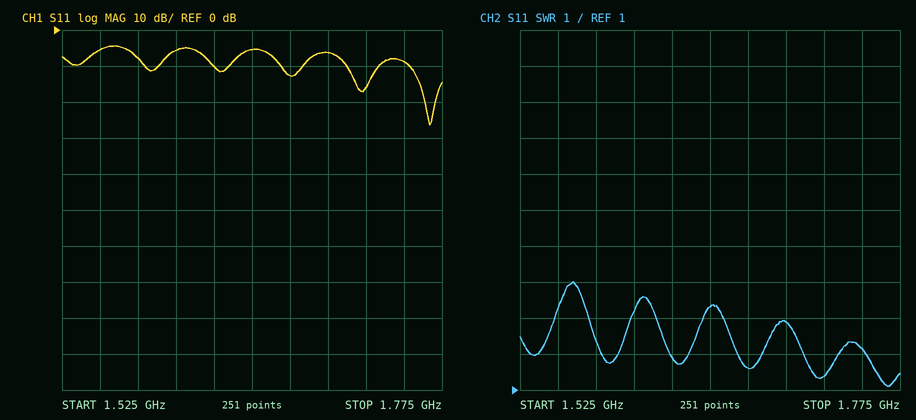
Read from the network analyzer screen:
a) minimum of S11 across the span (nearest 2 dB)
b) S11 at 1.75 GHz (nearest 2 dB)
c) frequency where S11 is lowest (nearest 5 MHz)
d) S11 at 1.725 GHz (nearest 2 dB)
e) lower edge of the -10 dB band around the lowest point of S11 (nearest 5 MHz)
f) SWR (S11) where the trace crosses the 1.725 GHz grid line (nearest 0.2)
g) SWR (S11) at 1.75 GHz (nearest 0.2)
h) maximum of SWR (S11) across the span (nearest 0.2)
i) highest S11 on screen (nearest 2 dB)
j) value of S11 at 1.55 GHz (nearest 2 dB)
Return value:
-26 dB
-8 dB
1.765 GHz
-16 dB
1.755 GHz
1.4
2.2
4.0
-4 dB
-6 dB
